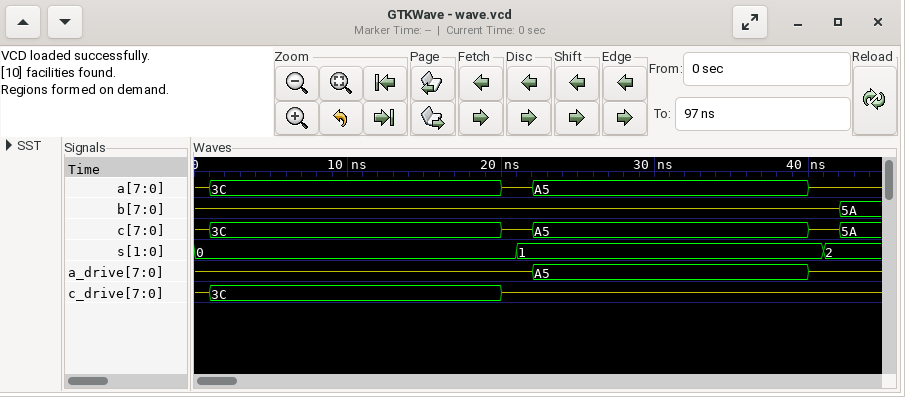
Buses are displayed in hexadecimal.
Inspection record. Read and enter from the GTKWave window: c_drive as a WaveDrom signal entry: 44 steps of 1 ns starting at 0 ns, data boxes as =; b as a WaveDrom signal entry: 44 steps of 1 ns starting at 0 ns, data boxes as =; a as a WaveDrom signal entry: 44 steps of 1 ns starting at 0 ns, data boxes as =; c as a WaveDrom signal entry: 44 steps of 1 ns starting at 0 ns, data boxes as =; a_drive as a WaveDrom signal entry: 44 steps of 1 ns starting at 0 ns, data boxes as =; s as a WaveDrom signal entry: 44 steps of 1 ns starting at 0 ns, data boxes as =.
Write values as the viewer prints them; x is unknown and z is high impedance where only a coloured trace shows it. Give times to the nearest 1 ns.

{name: 'c_drive', wave: 'z=..................z.......................', data: '3C'}
{name: 'b', wave: 'z.........................................=.', data: '5A'}
{name: 'a', wave: 'z=..................z.=.................z...', data: '3C A5'}
{name: 'c', wave: 'z=..................z.=.................z.=.', data: '3C A5 5A'}
{name: 'a_drive', wave: 'z.....................=.................z...', data: 'A5'}
{name: 's', wave: '=....................=...................=..', data: '0 1 2'}
